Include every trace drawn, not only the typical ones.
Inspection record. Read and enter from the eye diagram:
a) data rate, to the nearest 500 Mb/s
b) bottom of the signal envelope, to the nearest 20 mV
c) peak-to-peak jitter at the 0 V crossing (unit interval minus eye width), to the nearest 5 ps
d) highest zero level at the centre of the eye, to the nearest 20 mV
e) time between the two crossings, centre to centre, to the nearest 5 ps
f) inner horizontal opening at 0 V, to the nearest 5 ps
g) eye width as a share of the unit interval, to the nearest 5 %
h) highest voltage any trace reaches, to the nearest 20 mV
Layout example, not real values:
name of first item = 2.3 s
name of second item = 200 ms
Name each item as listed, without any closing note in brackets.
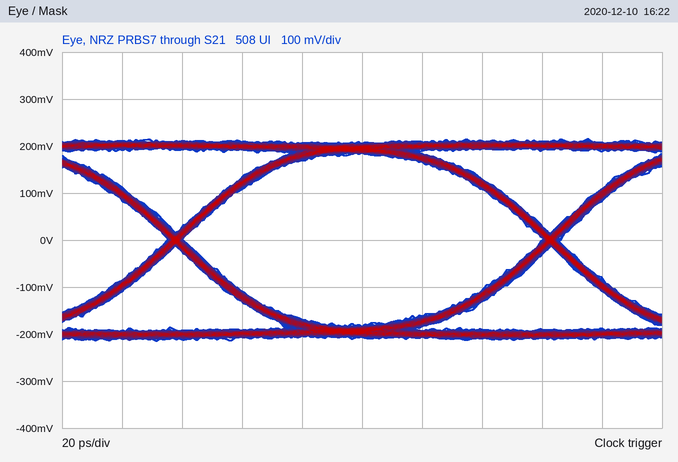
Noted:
data rate, to the nearest 500 Mb/s = 8.0 Gb/s
bottom of the signal envelope, to the nearest 20 mV = -220 mV
peak-to-peak jitter at the 0 V crossing (unit interval minus eye width), to the nearest 5 ps = 5 ps
highest zero level at the centre of the eye, to the nearest 20 mV = -180 mV
time between the two crossings, centre to centre, to the nearest 5 ps = 125 ps
inner horizontal opening at 0 V, to the nearest 5 ps = 120 ps
eye width as a share of the unit interval, to the nearest 5 % = 95 %
highest voltage any trace reaches, to the nearest 20 mV = 220 mV
